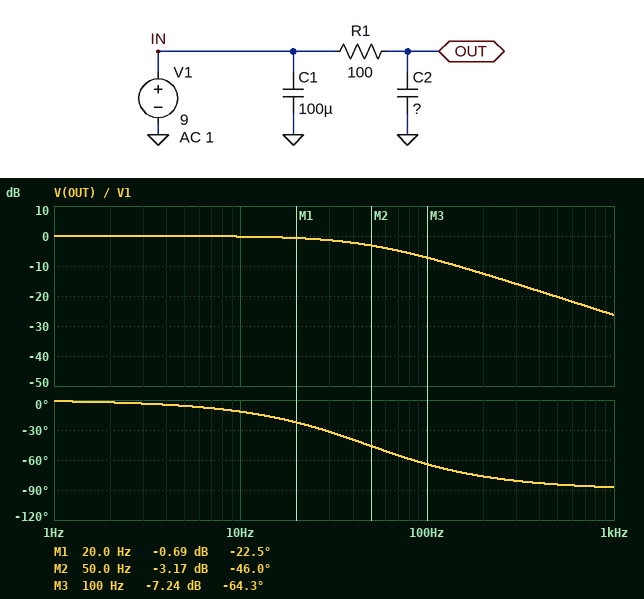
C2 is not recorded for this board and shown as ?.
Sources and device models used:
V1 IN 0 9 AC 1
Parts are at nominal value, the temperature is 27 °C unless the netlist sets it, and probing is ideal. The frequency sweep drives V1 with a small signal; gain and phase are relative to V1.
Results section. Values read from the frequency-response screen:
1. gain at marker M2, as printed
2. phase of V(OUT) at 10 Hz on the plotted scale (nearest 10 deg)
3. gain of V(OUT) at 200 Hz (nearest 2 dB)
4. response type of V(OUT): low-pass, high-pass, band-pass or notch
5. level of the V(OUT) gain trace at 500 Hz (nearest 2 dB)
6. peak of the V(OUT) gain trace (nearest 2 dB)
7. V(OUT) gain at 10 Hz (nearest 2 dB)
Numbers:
-3.17 dB
-10 deg
-12 dB
low-pass
-20 dB
0 dB
0 dB
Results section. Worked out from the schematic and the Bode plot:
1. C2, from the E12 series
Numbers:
33 µF
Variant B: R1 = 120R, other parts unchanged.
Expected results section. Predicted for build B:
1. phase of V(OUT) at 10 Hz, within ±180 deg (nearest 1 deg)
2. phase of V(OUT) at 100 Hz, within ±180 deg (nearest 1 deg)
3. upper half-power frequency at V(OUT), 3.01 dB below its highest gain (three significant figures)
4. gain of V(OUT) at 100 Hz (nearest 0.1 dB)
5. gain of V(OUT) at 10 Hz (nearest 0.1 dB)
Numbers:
-14 deg
-68 deg
40.2 Hz
-8.6 dB
-0.3 dB
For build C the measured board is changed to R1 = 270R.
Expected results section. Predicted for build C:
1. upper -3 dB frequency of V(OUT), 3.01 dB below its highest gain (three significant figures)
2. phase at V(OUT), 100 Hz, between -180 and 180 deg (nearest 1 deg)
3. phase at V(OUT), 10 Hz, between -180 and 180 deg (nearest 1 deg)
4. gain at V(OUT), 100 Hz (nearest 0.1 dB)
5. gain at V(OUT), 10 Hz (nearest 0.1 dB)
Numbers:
17.9 Hz
-80 deg
-29 deg
-15.1 dB
-1.2 dB
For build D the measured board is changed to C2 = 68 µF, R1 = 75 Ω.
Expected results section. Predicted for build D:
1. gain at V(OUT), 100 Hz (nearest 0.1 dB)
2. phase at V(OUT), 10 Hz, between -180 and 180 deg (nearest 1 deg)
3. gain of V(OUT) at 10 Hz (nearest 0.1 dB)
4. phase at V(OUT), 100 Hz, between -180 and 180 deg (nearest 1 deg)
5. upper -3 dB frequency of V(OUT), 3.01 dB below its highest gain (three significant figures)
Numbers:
-10.5 dB
-18 deg
-0.4 dB
-73 deg
31.2 Hz
